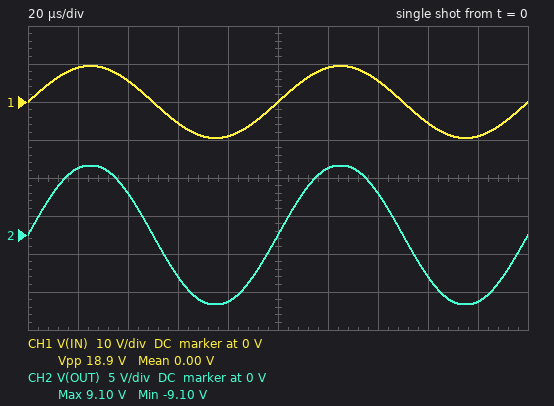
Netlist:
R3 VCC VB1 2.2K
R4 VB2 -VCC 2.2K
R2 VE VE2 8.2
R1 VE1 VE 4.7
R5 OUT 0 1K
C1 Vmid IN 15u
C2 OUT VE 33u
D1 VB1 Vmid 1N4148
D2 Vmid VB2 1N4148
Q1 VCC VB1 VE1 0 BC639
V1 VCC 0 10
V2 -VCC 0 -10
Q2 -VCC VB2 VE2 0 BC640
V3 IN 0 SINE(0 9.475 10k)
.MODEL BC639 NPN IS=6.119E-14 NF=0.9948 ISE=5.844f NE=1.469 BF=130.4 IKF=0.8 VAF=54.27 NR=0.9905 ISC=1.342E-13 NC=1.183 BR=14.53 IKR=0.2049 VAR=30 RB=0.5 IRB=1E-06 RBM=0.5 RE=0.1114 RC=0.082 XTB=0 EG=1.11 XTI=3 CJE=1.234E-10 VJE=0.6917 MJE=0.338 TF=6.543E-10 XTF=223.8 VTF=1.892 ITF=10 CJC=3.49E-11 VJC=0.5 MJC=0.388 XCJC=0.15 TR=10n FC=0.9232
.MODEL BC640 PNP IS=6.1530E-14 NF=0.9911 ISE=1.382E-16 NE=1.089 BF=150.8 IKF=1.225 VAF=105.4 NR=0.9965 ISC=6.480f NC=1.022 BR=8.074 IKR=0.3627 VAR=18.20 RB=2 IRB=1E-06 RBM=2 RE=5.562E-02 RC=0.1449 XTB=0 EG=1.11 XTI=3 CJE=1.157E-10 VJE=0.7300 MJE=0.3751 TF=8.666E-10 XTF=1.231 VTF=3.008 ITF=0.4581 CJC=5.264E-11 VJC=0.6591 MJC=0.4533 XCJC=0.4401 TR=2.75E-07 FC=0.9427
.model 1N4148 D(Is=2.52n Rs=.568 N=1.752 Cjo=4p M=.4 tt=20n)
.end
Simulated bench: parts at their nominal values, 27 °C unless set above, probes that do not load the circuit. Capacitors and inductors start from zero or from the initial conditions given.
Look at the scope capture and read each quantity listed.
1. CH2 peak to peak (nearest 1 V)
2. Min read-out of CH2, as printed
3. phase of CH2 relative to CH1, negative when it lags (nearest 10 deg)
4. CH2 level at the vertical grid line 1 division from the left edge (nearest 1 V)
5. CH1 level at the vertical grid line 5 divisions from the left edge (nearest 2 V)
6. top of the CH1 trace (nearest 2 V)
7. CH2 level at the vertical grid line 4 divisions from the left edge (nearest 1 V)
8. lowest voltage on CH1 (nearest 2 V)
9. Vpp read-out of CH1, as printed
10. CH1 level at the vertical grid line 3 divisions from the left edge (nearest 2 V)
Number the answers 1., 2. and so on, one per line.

1. 18 V
2. -9.10 V
3. 0 deg
4. 9 V
5. 0 V
6. 10 V
7. -9 V
8. -10 V
9. 18.9 V
10. -6 V
